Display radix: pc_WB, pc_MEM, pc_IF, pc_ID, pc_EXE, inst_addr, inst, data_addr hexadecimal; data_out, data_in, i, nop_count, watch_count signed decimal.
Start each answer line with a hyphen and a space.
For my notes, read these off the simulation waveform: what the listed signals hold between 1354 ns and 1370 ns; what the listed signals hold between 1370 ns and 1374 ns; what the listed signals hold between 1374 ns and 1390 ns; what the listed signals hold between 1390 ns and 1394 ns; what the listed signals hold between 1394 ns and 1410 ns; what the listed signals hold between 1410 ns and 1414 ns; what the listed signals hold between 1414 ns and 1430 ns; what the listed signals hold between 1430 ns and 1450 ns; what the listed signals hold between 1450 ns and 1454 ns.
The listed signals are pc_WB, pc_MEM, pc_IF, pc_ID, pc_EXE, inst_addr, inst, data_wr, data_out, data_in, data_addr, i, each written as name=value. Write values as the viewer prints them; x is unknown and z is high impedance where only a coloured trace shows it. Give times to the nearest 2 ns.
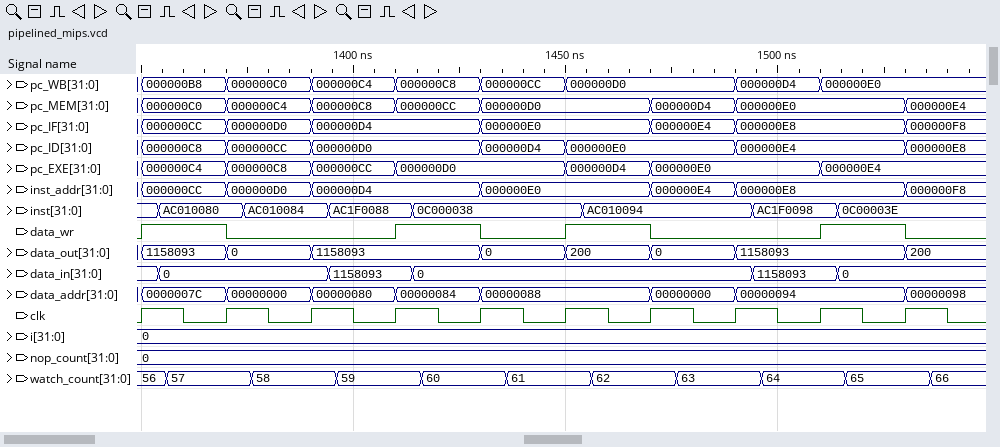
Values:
- pc_WB=000000B8, pc_MEM=000000C0, pc_IF=000000CC, pc_ID=000000C8, pc_EXE=000000C4, inst_addr=000000CC, inst=AC010080, data_wr=1, data_out=1158093, data_in=0, data_addr=0000007C, i=0
- pc_WB=000000C0, pc_MEM=000000C4, pc_IF=000000D0, pc_ID=000000CC, pc_EXE=000000C8, inst_addr=000000D0, inst=AC010080, data_wr=0, data_out=0, data_in=0, data_addr=00000000, i=0
- pc_WB=000000C0, pc_MEM=000000C4, pc_IF=000000D0, pc_ID=000000CC, pc_EXE=000000C8, inst_addr=000000D0, inst=AC010084, data_wr=0, data_out=0, data_in=0, data_addr=00000000, i=0
- pc_WB=000000C4, pc_MEM=000000C8, pc_IF=000000D4, pc_ID=000000D0, pc_EXE=000000CC, inst_addr=000000D4, inst=AC010084, data_wr=0, data_out=1158093, data_in=0, data_addr=00000080, i=0
- pc_WB=000000C4, pc_MEM=000000C8, pc_IF=000000D4, pc_ID=000000D0, pc_EXE=000000CC, inst_addr=000000D4, inst=AC1F0088, data_wr=0, data_out=1158093, data_in=1158093, data_addr=00000080, i=0
- pc_WB=000000C8, pc_MEM=000000CC, pc_IF=000000D4, pc_ID=000000D0, pc_EXE=000000D0, inst_addr=000000D4, inst=AC1F0088, data_wr=1, data_out=1158093, data_in=1158093, data_addr=00000084, i=0
- pc_WB=000000C8, pc_MEM=000000CC, pc_IF=000000D4, pc_ID=000000D0, pc_EXE=000000D0, inst_addr=000000D4, inst=0C000038, data_wr=1, data_out=1158093, data_in=0, data_addr=00000084, i=0
- pc_WB=000000CC, pc_MEM=000000D0, pc_IF=000000E0, pc_ID=000000D4, pc_EXE=000000D0, inst_addr=000000E0, inst=0C000038, data_wr=0, data_out=0, data_in=0, data_addr=00000088, i=0
- pc_WB=000000D0, pc_MEM=000000D0, pc_IF=000000E0, pc_ID=000000E0, pc_EXE=000000D4, inst_addr=000000E0, inst=0C000038, data_wr=1, data_out=200, data_in=0, data_addr=00000088, i=0
